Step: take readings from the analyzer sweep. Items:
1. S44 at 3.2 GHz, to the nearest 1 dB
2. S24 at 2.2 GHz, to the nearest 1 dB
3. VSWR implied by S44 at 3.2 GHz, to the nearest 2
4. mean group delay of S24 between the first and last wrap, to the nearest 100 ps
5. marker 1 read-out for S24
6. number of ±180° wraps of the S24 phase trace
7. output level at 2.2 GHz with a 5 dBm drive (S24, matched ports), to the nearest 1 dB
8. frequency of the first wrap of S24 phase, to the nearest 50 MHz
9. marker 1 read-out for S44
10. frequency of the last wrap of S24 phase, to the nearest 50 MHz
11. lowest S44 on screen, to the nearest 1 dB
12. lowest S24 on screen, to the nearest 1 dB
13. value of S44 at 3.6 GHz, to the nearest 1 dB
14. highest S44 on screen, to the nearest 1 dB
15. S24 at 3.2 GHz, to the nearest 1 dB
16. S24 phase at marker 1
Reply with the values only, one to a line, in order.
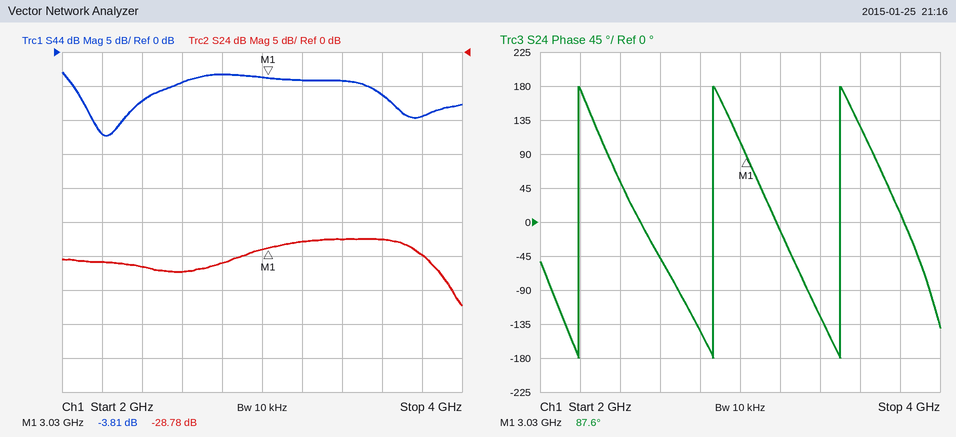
-4 dB
-31 dB
4
1.5 ns
-28.78 dB
3
-26 dBm
2.20 GHz
-3.81 dB
3.50 GHz
-12 dB
-37 dB
-6 dB
-3 dB
-28 dB
87.6°
